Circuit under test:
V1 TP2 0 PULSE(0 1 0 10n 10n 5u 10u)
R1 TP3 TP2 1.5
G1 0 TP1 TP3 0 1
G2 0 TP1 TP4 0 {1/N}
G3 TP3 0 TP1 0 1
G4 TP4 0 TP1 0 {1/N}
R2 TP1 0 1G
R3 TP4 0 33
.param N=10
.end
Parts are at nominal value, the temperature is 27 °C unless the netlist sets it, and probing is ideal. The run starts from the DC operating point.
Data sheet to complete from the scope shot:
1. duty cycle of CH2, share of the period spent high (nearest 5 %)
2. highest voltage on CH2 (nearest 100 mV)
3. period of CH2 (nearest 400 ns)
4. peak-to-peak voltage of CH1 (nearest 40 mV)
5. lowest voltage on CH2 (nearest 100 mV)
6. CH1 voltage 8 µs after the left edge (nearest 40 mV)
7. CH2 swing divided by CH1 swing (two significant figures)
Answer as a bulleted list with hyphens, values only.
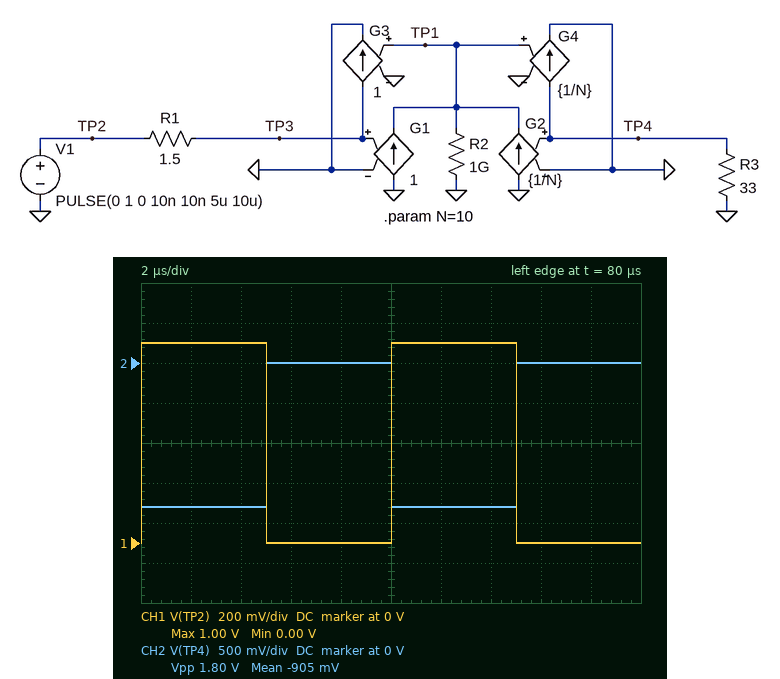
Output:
- 50 %
- 0 V
- 10.0 µs
- 1.00 V
- -1.8 V
- 0 V
- 1.8
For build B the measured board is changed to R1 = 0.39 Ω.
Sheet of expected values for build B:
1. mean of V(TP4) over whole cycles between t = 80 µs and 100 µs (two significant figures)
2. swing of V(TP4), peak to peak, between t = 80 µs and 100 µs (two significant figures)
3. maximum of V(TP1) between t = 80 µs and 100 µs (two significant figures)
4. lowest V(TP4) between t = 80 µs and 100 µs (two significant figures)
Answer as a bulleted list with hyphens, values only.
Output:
- -2.3 V
- 4.6 V
- 1.4 V
- -4.6 V
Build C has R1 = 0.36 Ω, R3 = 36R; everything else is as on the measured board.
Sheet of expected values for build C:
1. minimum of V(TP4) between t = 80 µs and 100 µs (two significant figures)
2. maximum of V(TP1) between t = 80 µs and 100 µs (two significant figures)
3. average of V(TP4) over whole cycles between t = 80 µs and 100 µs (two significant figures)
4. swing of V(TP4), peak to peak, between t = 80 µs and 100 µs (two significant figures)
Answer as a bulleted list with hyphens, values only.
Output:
- -5.0 V
- 1.4 V
- -2.5 V
- 5.0 V
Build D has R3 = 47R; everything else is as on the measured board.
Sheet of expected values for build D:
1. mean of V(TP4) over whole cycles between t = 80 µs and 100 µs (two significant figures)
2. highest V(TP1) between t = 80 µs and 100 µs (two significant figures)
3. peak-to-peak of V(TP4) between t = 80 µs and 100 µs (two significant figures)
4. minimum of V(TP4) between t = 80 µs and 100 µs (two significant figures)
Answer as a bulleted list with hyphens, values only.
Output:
- -1.2 V
- 510 mV
- 2.4 V
- -2.4 V
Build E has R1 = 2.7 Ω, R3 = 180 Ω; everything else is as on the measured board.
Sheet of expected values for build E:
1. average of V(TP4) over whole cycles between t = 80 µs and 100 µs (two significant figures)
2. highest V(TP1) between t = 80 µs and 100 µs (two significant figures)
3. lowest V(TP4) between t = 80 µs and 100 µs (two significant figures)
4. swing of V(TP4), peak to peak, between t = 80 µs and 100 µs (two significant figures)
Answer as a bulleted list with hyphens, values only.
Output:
- -2.0 V
- 220 mV
- -4.0 V
- 4.0 V
